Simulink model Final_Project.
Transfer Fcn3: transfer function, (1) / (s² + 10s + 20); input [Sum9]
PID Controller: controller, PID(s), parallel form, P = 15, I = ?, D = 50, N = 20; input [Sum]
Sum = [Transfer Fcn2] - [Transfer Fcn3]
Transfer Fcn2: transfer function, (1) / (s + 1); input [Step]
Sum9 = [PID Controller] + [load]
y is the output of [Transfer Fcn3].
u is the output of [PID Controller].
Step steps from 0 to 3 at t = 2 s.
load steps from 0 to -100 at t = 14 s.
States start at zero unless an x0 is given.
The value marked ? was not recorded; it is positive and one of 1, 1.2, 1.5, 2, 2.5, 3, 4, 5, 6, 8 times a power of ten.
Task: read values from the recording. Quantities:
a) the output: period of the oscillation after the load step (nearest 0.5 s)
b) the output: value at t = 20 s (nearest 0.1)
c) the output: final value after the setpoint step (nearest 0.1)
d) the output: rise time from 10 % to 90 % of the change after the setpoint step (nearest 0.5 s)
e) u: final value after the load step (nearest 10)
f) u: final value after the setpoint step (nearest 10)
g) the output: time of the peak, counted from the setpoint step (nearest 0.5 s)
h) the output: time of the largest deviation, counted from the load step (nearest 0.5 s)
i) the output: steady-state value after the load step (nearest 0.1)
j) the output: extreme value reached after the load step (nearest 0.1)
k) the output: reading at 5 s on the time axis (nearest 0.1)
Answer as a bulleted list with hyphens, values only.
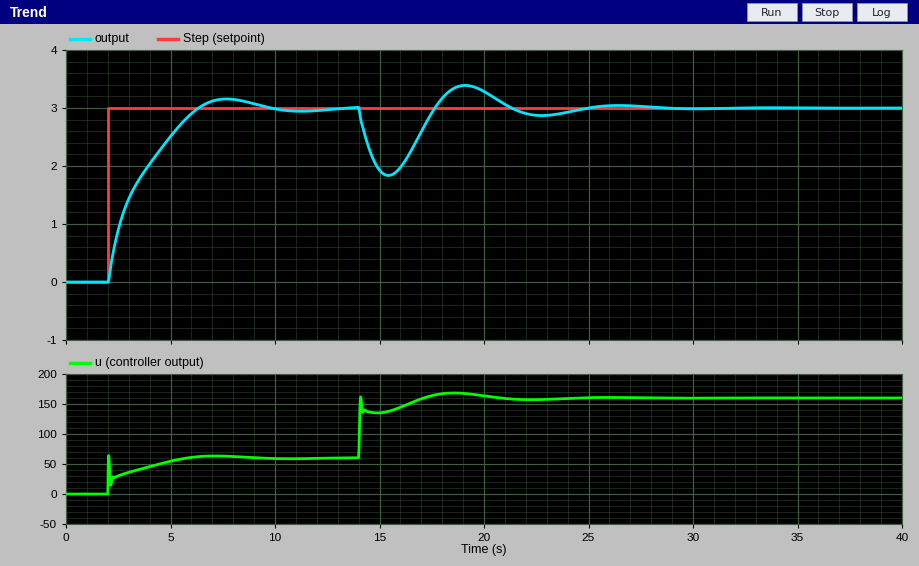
- 7.5 s
- 3.3
- 3.0
- 3.5 s
- 160
- 60
- 5.5 s
- 1.5 s
- 3.0
- 1.8
- 2.5
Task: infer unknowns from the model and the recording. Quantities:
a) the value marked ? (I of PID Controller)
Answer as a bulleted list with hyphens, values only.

- 50
